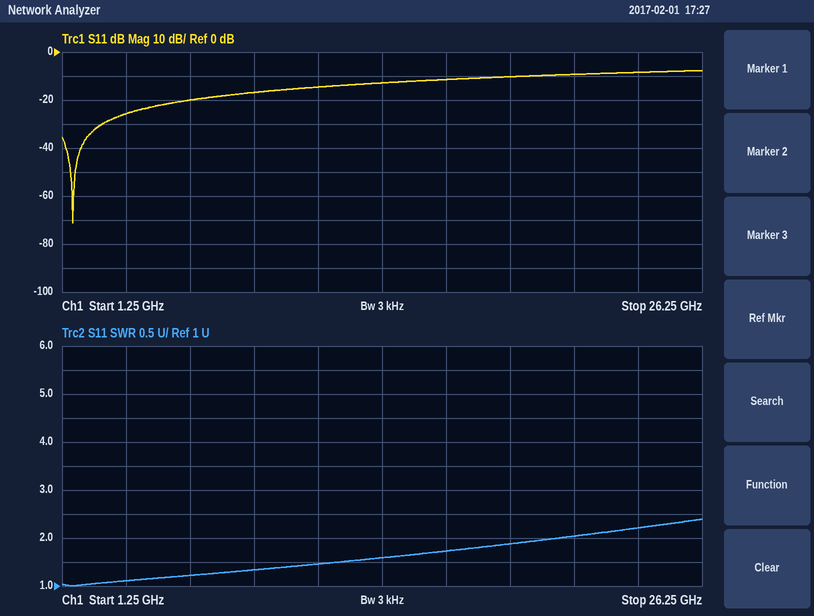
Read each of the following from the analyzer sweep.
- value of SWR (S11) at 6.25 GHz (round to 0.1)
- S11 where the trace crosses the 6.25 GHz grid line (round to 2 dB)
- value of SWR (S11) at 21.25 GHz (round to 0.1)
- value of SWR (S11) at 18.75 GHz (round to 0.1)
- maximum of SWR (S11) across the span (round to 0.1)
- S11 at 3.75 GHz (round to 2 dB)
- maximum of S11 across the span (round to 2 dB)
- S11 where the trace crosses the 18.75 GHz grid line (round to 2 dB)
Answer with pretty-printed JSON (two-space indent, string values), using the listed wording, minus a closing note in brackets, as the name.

{
  "value of SWR (S11) at 6.25 GHz": "1.2",
  "S11 where the trace crosses the 6.25 GHz grid line": "-20 dB",
  "value of SWR (S11) at 21.25 GHz": "2.0",
  "value of SWR (S11) at 18.75 GHz": "1.9",
  "maximum of SWR (S11) across the span": "2.4",
  "S11 at 3.75 GHz": "-26 dB",
  "maximum of S11 across the span": "-8 dB",
  "S11 where the trace crosses the 18.75 GHz grid line": "-10 dB"
}
